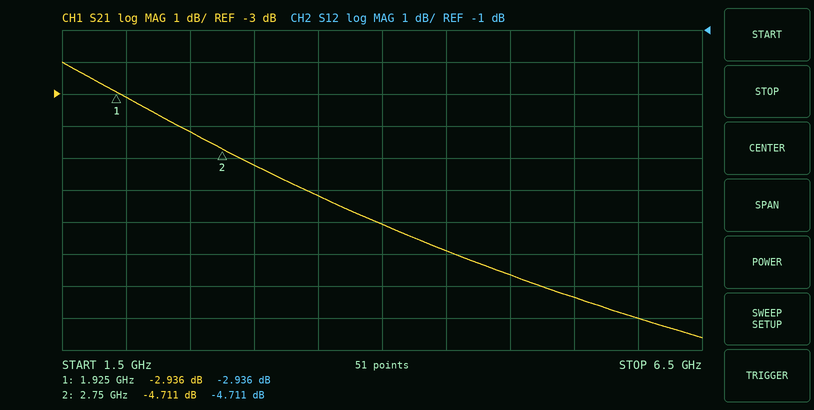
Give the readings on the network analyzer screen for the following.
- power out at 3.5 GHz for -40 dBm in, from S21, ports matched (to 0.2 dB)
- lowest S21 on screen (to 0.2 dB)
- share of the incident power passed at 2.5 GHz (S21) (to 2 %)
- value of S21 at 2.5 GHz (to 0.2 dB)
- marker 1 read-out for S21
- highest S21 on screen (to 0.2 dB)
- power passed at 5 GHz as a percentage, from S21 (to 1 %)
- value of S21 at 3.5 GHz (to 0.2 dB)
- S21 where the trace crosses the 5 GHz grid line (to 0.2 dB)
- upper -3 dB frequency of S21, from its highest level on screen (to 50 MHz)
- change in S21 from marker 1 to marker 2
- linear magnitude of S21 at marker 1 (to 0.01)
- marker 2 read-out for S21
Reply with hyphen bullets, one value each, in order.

- -46.2 dBm
- -10.6 dB
- 38 %
- -4.2 dB
- -2.936 dB
- -2.0 dB
- 14 %
- -6.2 dB
- -8.6 dB
- 2.90 GHz
- -1.775 dB
- 0.71
- -4.711 dB
